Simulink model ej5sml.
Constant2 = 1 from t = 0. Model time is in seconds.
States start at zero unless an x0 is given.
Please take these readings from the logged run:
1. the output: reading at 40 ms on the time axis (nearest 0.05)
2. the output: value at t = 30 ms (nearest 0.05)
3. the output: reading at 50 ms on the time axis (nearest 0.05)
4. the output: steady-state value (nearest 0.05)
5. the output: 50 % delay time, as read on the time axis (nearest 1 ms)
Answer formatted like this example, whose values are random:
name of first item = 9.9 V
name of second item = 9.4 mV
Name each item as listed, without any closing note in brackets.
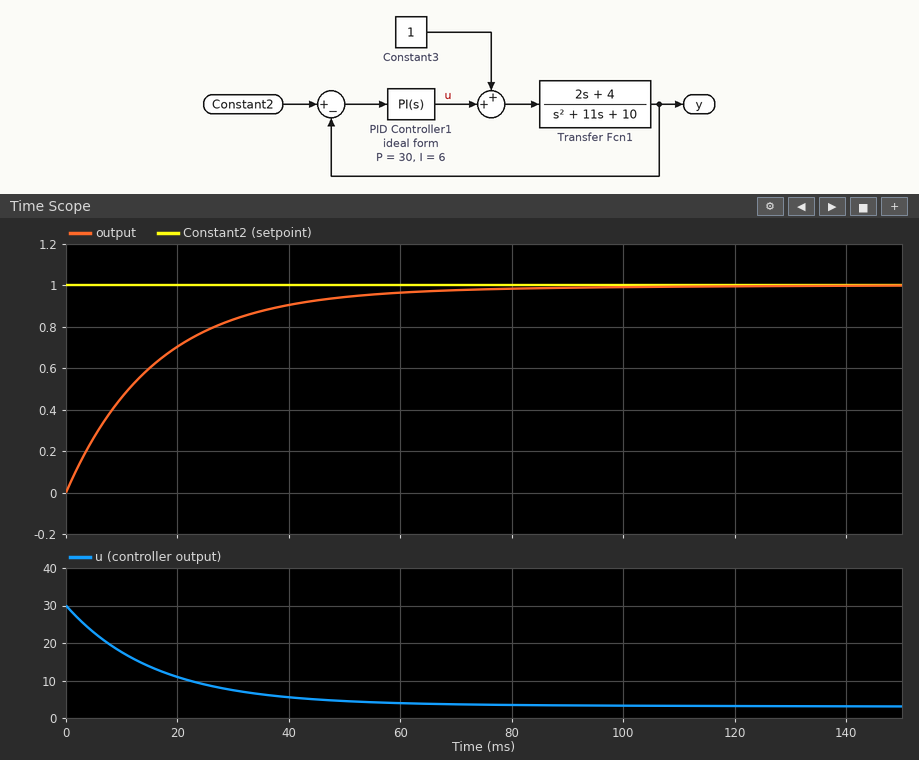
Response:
the output: reading at 40 ms on the time axis = 0.90
the output: value at t = 30 ms = 0.85
the output: reading at 50 ms on the time axis = 0.95
the output: steady-state value = 1.00
the output: 50 % delay time, as read on the time axis = 11 ms
